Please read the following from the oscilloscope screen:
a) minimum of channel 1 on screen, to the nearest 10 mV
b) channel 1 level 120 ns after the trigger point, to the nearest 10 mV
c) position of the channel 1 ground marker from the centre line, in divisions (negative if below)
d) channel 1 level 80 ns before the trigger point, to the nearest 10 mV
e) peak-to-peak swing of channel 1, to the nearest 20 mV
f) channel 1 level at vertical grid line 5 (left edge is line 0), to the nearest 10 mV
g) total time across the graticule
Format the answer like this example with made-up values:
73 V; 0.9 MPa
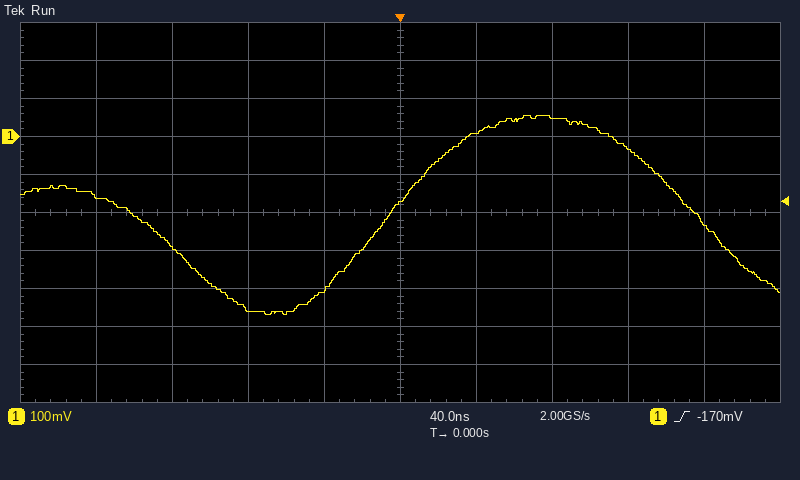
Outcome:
-470 mV; -30 mV; +2.0 div; -450 mV; 520 mV; -170 mV; 400 ns
